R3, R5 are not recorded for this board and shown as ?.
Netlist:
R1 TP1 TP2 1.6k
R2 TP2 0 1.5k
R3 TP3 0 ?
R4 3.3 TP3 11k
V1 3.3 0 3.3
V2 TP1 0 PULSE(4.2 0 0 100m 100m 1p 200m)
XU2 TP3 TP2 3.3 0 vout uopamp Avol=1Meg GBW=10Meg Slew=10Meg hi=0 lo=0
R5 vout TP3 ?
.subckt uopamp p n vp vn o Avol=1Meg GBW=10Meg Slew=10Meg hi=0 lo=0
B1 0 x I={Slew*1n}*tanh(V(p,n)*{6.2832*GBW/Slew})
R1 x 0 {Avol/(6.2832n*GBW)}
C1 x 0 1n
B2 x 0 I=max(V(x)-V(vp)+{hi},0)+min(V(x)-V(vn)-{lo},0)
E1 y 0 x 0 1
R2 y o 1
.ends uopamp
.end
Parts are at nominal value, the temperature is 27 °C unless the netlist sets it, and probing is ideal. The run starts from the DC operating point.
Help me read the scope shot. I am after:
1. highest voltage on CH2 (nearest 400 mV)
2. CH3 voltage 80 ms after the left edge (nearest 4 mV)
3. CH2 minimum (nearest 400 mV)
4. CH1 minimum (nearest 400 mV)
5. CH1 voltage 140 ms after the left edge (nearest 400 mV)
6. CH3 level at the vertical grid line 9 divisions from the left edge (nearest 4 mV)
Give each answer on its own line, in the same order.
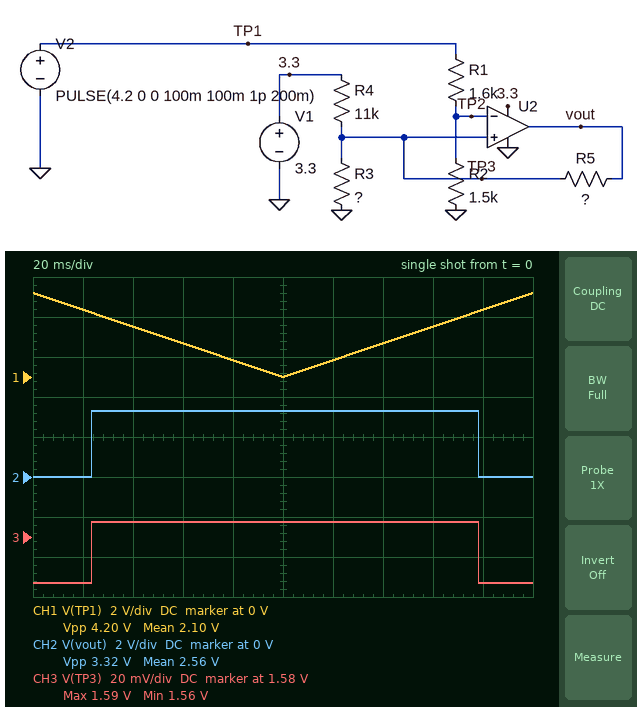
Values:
3.2 V
1.588 V
0 V
0 V
1.6 V
1.556 V
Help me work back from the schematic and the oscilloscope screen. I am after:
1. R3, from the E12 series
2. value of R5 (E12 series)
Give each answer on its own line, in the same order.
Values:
10 kΩ
560 kΩ
